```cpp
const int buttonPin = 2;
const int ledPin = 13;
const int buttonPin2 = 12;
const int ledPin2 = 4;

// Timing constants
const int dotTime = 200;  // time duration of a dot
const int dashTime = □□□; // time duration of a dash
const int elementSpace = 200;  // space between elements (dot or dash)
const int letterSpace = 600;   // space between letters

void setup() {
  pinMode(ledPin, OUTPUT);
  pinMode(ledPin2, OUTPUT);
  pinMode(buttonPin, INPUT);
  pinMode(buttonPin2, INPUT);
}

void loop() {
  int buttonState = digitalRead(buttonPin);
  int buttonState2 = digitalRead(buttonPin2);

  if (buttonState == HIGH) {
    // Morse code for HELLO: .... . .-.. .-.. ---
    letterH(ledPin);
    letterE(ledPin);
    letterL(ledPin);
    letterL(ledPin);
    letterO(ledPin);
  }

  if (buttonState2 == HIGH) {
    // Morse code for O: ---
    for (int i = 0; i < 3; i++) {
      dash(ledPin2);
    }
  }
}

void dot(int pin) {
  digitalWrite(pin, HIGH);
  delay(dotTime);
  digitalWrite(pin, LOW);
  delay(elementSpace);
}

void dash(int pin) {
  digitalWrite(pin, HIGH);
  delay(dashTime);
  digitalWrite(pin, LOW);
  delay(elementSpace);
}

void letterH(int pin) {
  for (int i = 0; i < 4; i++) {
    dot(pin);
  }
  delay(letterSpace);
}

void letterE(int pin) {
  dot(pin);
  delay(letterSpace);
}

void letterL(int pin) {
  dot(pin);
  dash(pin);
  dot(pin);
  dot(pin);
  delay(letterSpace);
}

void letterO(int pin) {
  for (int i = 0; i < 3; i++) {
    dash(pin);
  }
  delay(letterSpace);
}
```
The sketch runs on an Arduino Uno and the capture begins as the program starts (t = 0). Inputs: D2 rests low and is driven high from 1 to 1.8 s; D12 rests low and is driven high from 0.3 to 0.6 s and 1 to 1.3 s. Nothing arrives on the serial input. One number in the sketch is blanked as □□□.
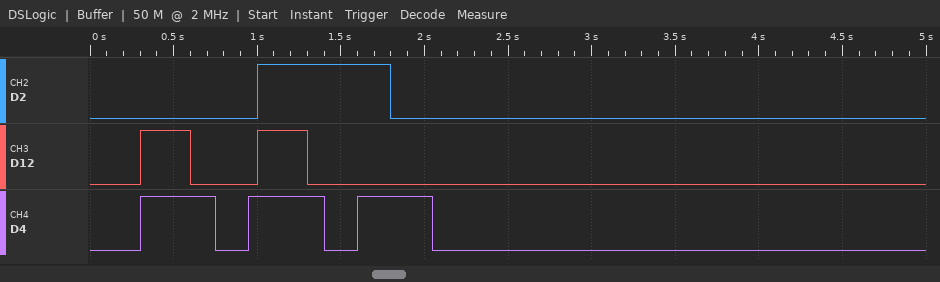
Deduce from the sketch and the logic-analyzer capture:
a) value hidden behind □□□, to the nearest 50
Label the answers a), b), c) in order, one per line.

a) 450
